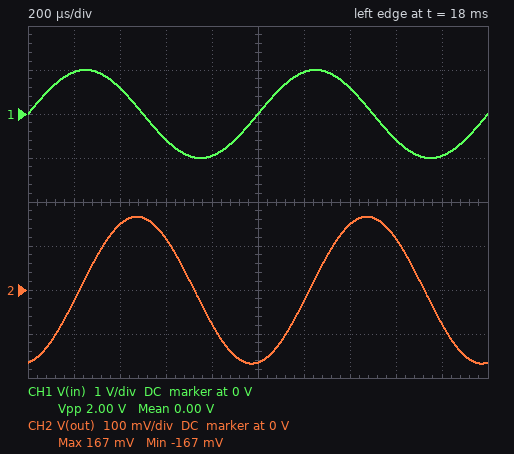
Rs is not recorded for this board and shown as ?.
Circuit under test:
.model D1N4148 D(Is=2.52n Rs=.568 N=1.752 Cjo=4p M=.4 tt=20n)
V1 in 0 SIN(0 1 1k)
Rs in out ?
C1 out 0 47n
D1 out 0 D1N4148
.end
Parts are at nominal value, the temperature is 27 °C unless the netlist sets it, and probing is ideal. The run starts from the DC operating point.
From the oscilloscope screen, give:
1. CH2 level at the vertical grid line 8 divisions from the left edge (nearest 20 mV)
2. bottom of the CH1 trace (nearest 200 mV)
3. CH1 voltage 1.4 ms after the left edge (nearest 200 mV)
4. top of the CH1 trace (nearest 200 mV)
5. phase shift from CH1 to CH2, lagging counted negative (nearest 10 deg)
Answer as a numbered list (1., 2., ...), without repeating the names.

1. 120 mV
2. -1.0 V
3. 600 mV
4. 1.0 V
5. -80 deg
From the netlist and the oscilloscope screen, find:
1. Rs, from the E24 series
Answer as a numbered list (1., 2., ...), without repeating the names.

1. 20 kΩ
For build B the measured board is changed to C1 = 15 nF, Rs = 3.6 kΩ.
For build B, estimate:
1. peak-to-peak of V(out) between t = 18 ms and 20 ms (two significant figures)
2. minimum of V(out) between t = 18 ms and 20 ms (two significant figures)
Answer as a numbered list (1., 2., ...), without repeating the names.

1. 1.4 V
2. -950 mV
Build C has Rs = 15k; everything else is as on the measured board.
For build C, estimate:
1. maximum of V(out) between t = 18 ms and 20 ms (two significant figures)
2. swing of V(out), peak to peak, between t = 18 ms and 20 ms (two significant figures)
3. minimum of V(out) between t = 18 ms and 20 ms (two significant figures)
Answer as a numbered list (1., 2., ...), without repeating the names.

1. 220 mV
2. 440 mV
3. -220 mV
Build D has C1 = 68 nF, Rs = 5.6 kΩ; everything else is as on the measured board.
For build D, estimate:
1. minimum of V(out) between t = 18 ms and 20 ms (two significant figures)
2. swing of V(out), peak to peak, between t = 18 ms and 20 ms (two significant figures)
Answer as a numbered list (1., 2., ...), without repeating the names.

1. -390 mV
2. 770 mV
